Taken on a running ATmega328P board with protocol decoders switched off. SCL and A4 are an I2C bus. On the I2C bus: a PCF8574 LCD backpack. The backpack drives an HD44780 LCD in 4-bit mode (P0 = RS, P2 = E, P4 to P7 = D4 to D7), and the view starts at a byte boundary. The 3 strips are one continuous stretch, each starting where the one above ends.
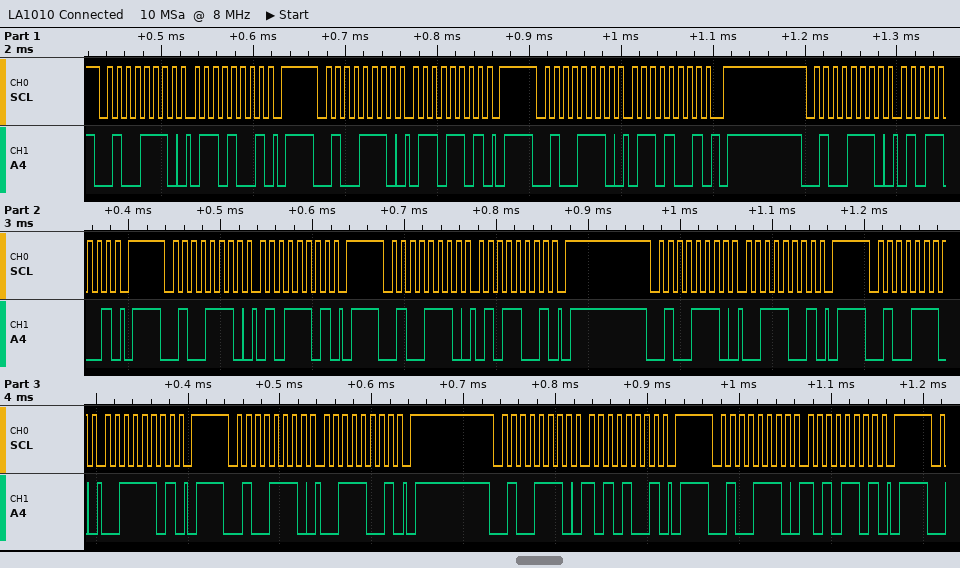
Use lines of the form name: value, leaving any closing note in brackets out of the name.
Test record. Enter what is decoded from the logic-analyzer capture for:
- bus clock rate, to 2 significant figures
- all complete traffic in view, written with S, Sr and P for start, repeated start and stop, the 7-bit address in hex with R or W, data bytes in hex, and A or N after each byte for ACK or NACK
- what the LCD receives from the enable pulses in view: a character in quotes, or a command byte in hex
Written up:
bus clock rate, to 2 significant figures: 100 kHz
all complete traffic in view, written with S, Sr and P for start, repeated start and stop, the 7-bit address in hex with R or W, data bytes in hex, and A or N after each byte for ACK or NACK: S 27W A 69 A P S 27W A 6D A P S 27W A 69 A P S 27W A 59 A P S 27W A 5D A P S 27W A 59 A P S 27W A 39 A P S 27W A 3D A P S 27W A 39 A P S 27W A A9 A P S 27W A AD A P
what the LCD receives from the enable pulses in view: a character in quotes, or a command byte in hex: 'e'
